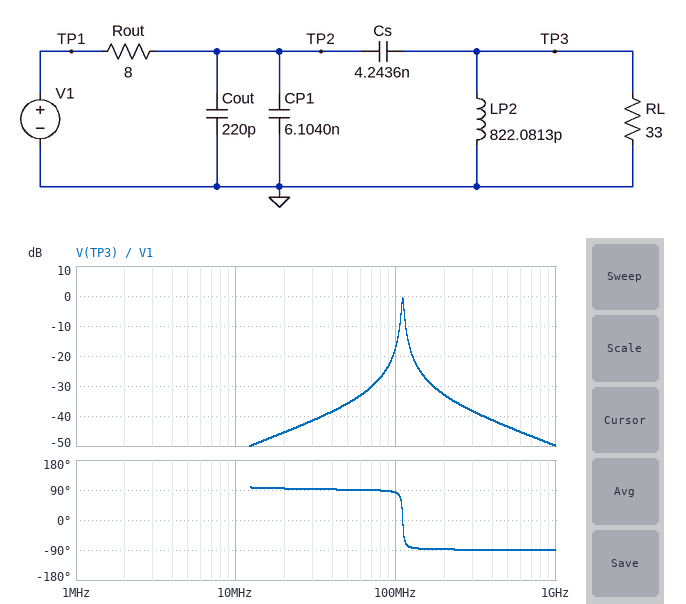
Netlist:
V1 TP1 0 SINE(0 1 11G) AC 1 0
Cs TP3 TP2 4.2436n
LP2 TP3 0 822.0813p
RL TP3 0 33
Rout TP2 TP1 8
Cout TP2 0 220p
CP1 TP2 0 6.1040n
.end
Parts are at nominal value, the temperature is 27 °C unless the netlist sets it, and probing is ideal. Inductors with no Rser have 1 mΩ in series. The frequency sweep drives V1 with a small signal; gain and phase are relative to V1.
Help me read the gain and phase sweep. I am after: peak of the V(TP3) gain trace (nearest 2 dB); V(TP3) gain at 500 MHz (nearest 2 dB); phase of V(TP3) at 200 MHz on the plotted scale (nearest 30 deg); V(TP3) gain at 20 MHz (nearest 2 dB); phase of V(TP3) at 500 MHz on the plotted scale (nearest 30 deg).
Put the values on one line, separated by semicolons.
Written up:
0 dB; -44 dB; -90 deg; -46 dB; -90 deg
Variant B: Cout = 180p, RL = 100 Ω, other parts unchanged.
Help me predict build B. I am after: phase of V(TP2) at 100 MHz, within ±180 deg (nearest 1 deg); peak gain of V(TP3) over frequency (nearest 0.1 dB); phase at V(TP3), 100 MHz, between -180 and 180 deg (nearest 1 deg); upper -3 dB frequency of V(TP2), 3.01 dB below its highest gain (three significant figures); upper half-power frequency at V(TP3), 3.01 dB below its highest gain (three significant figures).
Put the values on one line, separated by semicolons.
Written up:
84 deg; 3.6 dB; 85 deg; 1.89 MHz; 111 MHz
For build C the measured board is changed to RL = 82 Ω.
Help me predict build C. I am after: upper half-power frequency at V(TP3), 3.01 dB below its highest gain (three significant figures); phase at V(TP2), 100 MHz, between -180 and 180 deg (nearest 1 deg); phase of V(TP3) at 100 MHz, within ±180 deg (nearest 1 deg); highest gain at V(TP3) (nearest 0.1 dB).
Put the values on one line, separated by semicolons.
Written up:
111 MHz; 84 deg; 85 deg; 3.0 dB
